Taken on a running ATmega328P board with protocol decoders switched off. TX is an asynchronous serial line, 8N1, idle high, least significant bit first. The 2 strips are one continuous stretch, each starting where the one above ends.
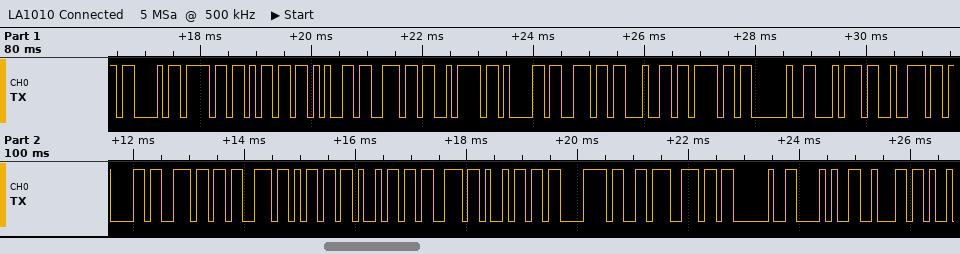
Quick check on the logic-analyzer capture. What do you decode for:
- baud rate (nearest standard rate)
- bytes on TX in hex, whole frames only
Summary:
9600 baud
43 6F 6D 65 6E 7A 61 6E 64 6F 20 74 72 61 6E 73 6D 69 73 69 C3 B3 6E 20 28 62
